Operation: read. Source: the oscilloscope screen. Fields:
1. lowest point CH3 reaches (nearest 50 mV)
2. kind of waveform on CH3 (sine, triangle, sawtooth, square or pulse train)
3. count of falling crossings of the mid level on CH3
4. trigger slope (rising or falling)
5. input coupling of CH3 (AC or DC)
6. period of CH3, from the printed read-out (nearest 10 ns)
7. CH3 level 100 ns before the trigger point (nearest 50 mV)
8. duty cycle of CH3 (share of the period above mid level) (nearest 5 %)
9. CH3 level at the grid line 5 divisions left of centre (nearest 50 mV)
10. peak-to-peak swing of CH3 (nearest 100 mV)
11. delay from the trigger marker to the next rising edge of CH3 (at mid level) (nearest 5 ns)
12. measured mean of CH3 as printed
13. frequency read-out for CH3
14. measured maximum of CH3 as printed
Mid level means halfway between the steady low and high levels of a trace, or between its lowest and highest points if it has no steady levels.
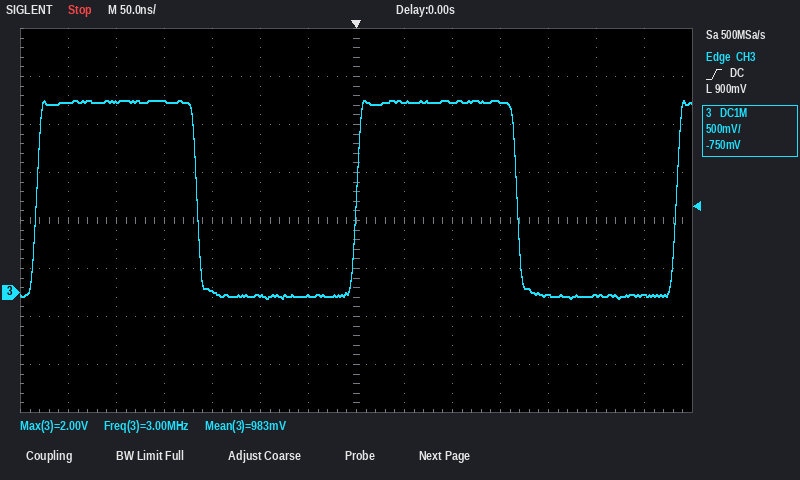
-50 mV
square
2
rising
DC
330 ns
-50 mV
50 %
2.00 V
2.10 V
335 ns
983 mV
3.00 MHz
2.00 V
